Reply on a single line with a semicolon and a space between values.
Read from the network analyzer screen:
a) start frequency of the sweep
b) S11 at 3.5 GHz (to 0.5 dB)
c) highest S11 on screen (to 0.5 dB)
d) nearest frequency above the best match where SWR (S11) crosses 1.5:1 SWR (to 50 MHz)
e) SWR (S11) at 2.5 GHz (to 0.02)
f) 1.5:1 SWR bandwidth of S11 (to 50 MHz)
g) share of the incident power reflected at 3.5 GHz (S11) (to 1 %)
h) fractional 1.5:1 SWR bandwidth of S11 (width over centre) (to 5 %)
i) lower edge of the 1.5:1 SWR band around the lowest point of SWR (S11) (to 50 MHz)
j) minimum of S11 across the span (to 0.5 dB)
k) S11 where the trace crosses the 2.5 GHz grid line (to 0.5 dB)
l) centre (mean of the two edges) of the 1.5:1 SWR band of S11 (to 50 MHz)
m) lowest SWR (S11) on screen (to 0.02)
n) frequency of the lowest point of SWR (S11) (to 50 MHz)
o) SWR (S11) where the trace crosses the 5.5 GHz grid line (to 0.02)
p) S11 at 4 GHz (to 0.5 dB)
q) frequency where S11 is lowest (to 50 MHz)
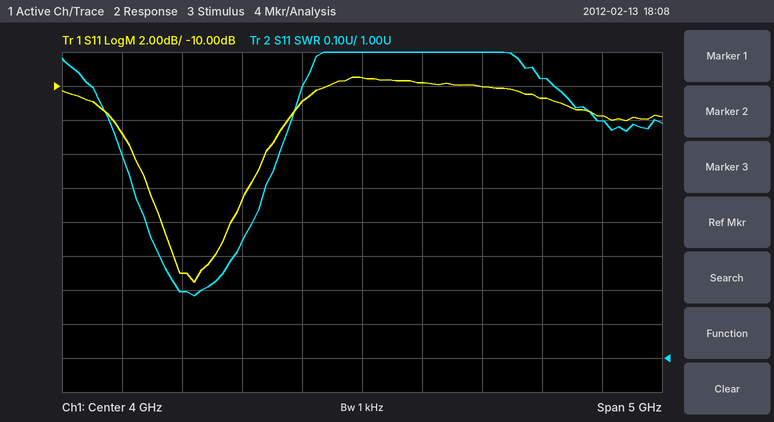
1.5 GHz; -11.0 dB; -9.5 dB; 3.20 GHz; 1.20; 1.10 GHz; 8 %; 40 %; 2.10 GHz; -21.5 dB; -21.0 dB; 2.65 GHz; 1.18; 2.60 GHz; 1.82; -9.5 dB; 2.60 GHz
